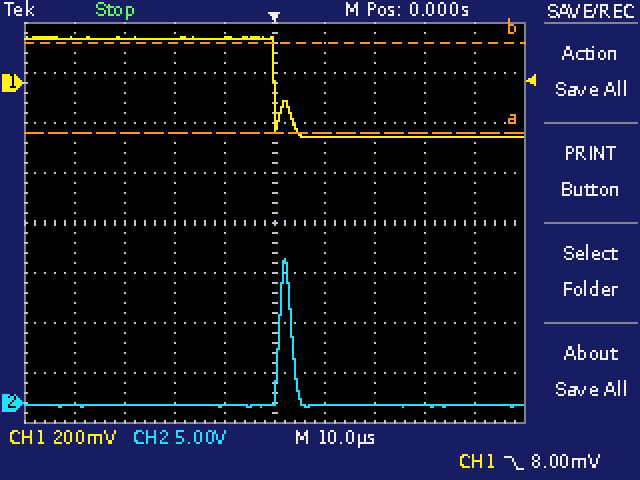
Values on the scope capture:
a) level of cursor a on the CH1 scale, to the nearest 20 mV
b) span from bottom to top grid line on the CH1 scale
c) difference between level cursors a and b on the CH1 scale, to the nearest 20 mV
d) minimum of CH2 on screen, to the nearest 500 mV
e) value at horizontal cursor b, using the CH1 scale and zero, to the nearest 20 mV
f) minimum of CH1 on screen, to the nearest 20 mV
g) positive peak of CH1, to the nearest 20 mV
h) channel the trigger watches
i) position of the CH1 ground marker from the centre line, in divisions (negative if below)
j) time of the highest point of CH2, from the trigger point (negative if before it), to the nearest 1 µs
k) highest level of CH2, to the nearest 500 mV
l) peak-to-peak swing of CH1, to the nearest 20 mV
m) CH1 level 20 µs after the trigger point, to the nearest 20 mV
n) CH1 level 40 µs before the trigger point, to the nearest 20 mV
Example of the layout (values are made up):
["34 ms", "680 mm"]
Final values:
["-200 mV", "1.6 V", "360 mV", "-500 mV", "160 mV", "-220 mV", "180 mV", "CH1", "+2.8 div", "+2 µs", "14.5 V", "400 mV", "-220 mV", "180 mV"]
